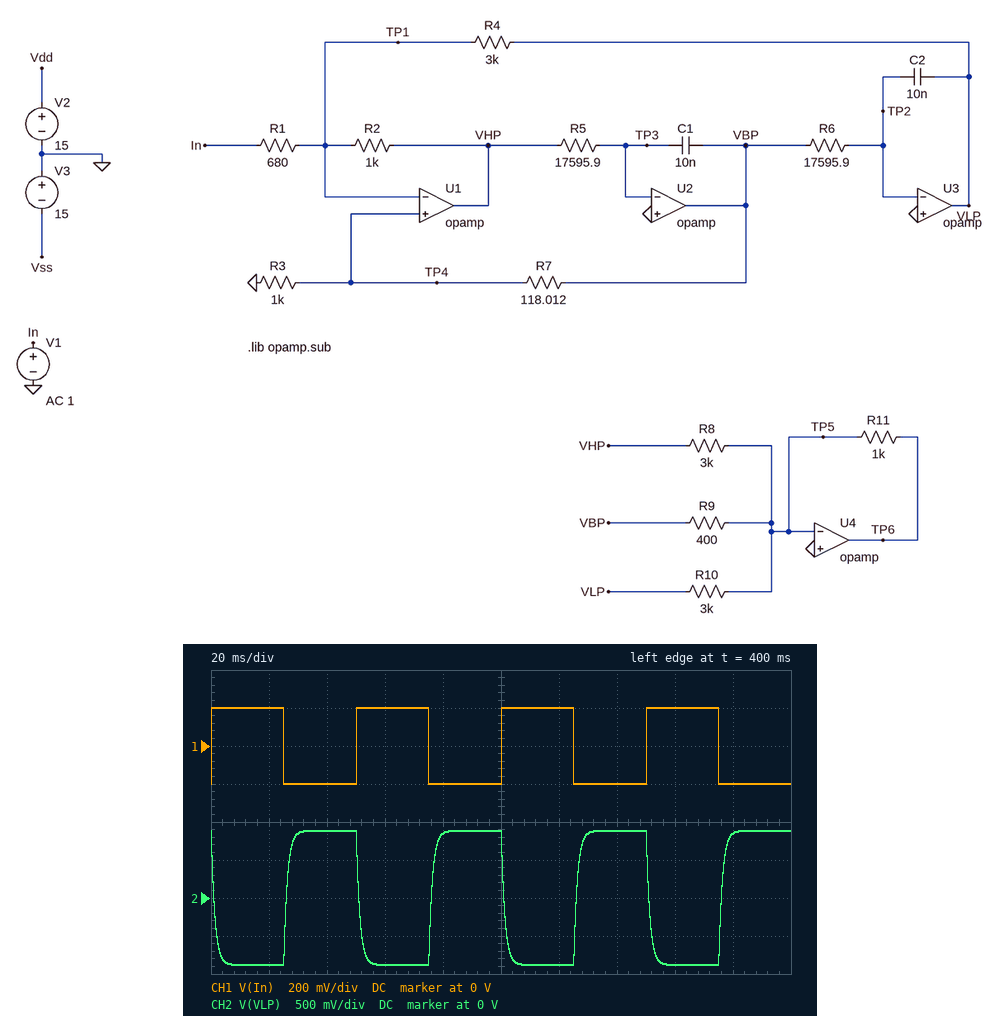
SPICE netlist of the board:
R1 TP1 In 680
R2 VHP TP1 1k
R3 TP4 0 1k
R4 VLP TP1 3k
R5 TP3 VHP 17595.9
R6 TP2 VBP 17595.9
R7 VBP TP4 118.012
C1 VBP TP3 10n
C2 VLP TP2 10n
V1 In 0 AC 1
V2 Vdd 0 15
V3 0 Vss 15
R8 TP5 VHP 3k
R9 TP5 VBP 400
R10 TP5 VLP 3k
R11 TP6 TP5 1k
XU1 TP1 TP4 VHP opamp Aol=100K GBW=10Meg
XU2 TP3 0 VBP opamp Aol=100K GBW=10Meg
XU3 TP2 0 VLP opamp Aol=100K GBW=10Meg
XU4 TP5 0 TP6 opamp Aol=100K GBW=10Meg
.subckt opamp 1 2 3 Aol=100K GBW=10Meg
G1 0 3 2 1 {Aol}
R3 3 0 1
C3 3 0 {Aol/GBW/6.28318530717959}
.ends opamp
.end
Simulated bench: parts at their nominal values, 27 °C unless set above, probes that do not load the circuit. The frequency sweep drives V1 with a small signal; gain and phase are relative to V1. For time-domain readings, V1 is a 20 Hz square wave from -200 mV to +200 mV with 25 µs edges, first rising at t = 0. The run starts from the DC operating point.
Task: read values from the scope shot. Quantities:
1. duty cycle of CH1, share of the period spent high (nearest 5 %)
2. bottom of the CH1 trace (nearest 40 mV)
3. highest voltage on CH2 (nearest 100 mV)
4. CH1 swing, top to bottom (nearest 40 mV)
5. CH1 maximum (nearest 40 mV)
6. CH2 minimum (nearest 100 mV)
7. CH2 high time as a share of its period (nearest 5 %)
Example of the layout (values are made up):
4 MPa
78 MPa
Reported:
50 %
-200 mV
900 mV
400 mV
200 mV
-900 mV
50 %
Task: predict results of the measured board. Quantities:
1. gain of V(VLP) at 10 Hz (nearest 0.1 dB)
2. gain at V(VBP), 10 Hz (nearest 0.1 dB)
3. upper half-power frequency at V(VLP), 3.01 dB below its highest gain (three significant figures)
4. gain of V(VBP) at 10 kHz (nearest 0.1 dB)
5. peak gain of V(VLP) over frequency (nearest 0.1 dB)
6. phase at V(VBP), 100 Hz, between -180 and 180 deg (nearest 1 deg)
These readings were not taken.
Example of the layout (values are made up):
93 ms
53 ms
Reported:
12.9 dB
-26.3 dB
127 Hz
-17.7 dB
12.9 dB
49 deg
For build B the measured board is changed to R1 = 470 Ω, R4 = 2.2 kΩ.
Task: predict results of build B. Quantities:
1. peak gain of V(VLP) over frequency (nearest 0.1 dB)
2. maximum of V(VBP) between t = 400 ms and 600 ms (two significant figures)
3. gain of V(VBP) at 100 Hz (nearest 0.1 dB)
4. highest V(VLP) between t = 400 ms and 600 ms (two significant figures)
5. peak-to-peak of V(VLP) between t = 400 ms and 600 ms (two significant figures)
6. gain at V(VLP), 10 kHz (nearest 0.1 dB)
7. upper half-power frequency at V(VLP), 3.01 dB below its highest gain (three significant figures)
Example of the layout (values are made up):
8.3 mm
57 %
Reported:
13.4 dB
240 mV
-7.6 dB
940 mV
1.9 V
-35.5 dB
134 Hz
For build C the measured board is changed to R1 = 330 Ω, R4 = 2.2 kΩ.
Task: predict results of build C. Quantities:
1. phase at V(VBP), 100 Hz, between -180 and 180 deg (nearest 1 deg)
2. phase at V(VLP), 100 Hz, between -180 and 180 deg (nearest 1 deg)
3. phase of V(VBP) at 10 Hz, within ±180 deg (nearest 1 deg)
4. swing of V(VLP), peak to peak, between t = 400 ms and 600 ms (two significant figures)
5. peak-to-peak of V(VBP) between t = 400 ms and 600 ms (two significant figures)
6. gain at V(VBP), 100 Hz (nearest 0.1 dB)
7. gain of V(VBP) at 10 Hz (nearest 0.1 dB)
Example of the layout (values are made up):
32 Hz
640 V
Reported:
45 deg
135 deg
84 deg
2.7 V
560 mV
-5.4 dB
-22.7 dB
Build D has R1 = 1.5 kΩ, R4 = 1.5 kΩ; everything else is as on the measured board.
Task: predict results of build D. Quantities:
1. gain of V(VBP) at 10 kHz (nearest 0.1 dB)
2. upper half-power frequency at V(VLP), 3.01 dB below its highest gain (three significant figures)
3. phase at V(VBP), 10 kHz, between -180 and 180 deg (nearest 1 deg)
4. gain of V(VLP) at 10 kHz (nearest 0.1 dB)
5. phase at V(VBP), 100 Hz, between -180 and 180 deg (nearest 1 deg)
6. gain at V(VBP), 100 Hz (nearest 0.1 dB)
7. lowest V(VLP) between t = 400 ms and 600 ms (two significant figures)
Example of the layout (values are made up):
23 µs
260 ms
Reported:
-24.5 dB
339 Hz
-79 deg
-45.4 dB
71 deg
-19.5 dB
-200 mV
